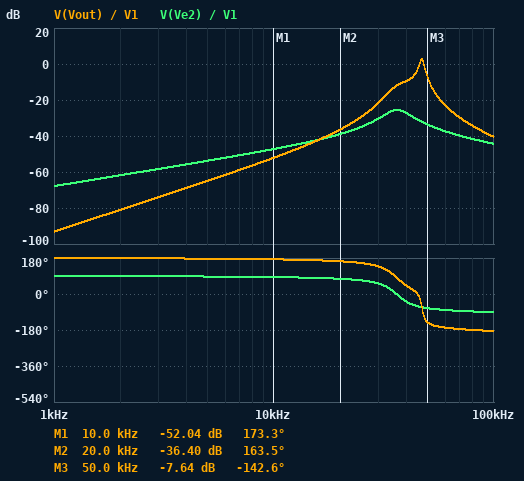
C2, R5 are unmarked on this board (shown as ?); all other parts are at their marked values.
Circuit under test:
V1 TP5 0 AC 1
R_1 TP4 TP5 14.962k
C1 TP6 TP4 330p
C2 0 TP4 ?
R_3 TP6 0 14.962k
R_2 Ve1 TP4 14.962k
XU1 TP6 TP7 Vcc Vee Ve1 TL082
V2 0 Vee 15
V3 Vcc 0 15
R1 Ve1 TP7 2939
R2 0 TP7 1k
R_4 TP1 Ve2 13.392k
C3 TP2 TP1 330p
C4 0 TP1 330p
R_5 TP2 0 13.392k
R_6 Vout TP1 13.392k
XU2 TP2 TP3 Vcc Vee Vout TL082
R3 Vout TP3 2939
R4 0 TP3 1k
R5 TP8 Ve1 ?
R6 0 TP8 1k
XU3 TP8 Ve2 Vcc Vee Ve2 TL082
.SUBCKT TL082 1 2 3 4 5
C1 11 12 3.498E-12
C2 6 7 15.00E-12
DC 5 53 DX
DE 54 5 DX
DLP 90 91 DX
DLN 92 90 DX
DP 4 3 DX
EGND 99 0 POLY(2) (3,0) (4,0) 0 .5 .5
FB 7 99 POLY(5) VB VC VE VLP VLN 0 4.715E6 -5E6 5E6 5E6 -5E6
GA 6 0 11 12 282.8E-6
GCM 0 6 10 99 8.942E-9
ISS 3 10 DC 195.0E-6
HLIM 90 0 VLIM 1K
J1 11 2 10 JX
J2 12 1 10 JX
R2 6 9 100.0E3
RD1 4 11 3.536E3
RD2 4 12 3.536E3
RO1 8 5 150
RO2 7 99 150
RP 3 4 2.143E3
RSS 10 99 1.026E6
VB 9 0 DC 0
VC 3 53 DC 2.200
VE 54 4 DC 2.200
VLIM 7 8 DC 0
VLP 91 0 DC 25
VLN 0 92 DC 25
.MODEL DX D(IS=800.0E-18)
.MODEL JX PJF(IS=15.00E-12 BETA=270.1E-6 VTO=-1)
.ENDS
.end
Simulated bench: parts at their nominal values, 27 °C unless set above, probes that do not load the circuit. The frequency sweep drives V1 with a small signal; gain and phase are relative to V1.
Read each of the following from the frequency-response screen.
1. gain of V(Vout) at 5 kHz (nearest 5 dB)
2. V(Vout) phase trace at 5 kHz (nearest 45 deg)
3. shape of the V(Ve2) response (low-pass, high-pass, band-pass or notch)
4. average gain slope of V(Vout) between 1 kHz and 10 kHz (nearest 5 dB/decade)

-65 dB
180 deg
band-pass
40 dB/decade
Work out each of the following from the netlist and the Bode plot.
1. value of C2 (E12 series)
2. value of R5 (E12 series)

470 pF
150 kΩ
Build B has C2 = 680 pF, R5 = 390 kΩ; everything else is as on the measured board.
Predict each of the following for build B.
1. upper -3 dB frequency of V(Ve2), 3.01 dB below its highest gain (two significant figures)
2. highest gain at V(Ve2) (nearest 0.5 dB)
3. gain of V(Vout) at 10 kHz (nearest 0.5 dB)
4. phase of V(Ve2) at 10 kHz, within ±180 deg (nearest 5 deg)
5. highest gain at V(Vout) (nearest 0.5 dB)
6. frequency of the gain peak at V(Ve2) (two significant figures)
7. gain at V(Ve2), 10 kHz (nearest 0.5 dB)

40 kHz
-41.0 dB
-60.0 dB
80 deg
-12.0 dB
31 kHz
-55.5 dB
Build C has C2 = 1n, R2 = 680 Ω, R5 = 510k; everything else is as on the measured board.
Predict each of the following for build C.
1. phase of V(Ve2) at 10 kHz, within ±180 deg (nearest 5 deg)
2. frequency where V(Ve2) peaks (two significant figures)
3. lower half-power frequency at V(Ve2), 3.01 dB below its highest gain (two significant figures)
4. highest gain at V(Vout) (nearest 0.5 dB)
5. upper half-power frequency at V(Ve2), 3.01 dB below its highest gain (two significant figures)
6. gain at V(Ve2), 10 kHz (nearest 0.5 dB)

80 deg
25 kHz
22 kHz
-16.0 dB
29 kHz
-54.5 dB
